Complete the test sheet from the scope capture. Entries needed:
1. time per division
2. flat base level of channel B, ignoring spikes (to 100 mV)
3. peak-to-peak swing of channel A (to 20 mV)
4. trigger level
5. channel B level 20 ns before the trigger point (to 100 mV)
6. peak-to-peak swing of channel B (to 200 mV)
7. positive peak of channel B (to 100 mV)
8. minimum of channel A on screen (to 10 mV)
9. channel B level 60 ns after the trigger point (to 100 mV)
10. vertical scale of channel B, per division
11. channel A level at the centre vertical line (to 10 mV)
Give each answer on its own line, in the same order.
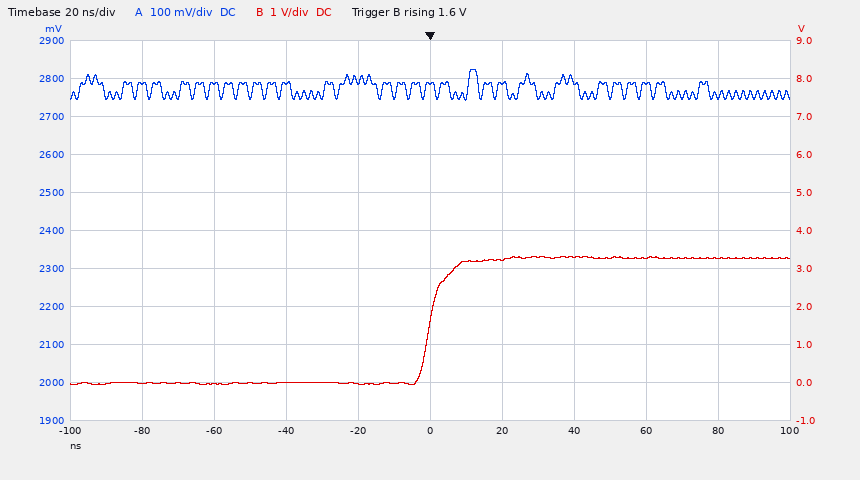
20 ns
0.0 V
80 mV
1.6 V
0.0 V
3.4 V
3.3 V
2.74 V
3.3 V
1 V
2.79 V
